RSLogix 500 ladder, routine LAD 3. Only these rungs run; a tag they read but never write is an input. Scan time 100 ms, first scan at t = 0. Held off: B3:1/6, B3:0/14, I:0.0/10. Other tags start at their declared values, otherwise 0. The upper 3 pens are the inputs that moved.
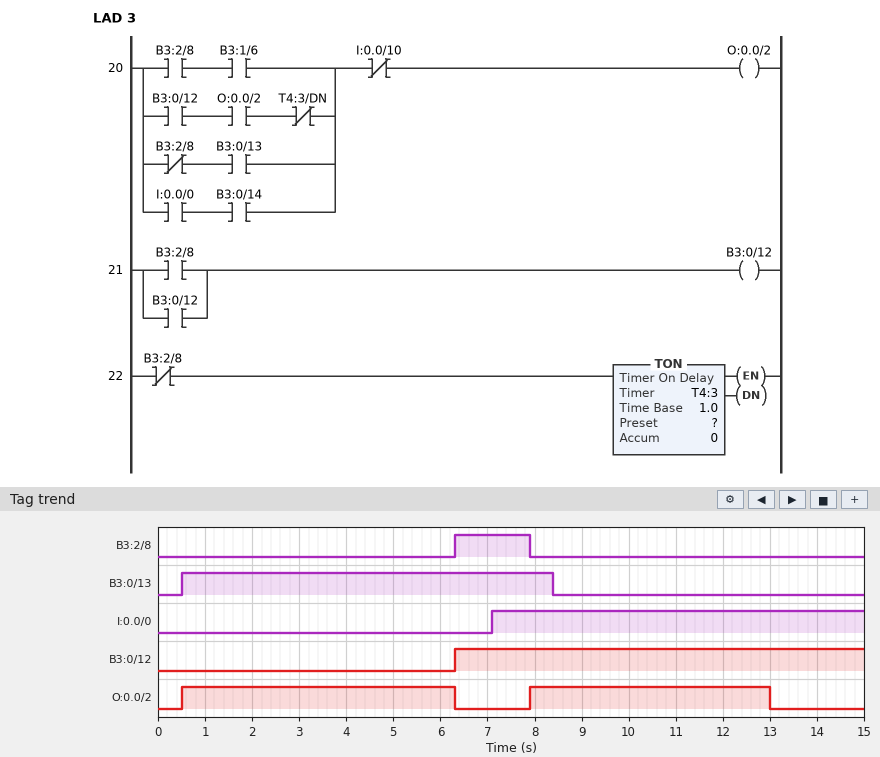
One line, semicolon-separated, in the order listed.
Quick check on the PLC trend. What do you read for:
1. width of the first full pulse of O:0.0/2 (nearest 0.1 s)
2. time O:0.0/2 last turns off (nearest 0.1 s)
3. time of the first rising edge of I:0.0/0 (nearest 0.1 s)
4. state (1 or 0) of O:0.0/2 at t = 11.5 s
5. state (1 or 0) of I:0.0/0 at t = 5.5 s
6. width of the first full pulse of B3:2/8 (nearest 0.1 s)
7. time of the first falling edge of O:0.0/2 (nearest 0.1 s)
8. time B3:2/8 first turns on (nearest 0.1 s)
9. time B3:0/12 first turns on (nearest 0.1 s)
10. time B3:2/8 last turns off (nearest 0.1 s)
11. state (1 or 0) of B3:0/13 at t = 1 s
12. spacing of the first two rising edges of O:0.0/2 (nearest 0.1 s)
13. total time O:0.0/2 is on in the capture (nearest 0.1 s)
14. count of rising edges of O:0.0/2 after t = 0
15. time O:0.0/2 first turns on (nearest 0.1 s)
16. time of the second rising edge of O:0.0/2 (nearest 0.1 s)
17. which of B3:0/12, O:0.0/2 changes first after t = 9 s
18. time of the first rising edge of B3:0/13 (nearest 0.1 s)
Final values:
5.8 s; 13.0 s; 7.1 s; 1; 0; 1.6 s; 6.3 s; 6.3 s; 6.3 s; 7.9 s; 1; 7.4 s; 10.9 s; 2; 0.5 s; 7.9 s; O:0.0/2; 0.5 s
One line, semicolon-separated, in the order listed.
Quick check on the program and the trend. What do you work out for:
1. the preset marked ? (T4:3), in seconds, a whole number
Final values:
5 s
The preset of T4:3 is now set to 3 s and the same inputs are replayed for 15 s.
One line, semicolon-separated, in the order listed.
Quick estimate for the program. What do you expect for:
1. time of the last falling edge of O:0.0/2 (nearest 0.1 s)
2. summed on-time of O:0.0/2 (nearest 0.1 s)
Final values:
11.0 s; 8.9 s
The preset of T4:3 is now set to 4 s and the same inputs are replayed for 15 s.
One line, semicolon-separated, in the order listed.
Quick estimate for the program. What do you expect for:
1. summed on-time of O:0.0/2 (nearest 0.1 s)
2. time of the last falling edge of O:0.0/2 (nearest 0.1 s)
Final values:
9.9 s; 12.0 s
